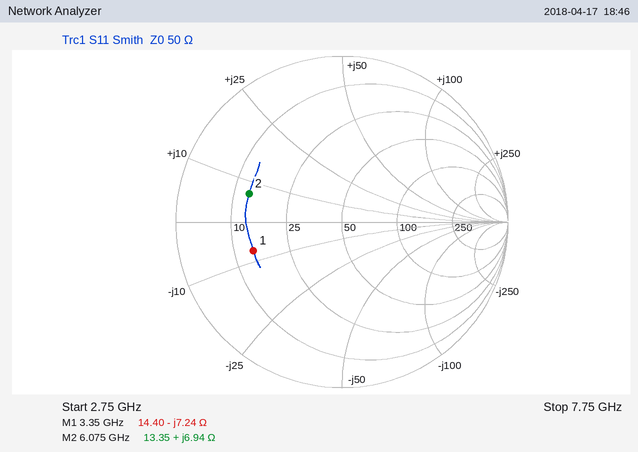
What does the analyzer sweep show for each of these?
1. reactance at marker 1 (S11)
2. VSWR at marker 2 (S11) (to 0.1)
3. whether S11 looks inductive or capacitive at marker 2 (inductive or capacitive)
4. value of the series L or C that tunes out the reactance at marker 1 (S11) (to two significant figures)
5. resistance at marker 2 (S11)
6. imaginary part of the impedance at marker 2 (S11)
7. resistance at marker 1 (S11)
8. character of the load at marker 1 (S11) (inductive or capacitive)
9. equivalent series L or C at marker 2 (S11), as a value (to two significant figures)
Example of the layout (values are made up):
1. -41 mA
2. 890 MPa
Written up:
1. -7.24 Ω
2. 3.8
3. inductive
4. 340 pH
5. 13.35 Ω
6. +6.94 Ω
7. 14.40 Ω
8. capacitive
9. 180 pH
